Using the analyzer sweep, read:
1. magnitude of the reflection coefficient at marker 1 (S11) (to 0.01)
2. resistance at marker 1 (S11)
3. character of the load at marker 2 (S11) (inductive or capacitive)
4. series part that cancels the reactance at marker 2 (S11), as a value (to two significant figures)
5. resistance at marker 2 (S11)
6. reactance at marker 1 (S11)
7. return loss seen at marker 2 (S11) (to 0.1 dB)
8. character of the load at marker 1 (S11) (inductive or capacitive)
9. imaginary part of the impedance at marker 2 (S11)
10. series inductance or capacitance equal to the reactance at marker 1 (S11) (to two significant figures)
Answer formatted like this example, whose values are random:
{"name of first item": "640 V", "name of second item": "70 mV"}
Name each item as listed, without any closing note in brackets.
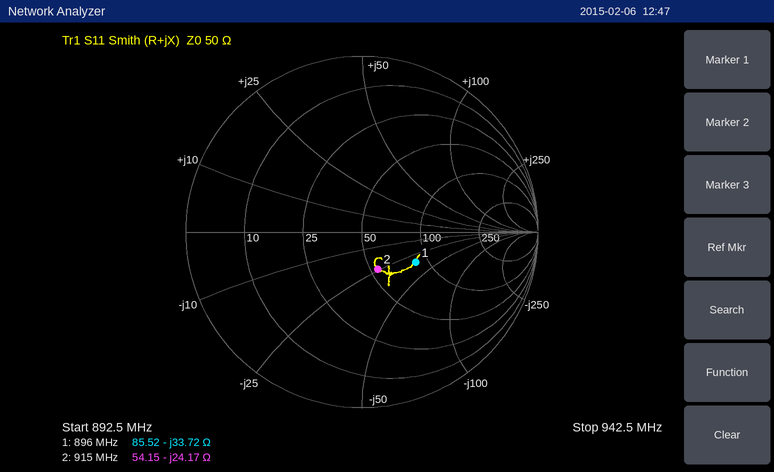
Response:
{"magnitude of the reflection coefficient at marker 1 (S11)": "0.35", "resistance at marker 1": "85.52 Ω", "character of the load at marker 2 (S11)": "capacitive", "series part that cancels the reactance at marker 2 (S11), as a value": "4.2 nH", "resistance at marker 2": "54.15 Ω", "reactance at marker 1": "-33.72 Ω", "return loss seen at marker 2 (S11)": "12.8 dB", "character of the load at marker 1 (S11)": "capacitive", "imaginary part of the impedance at marker 2": "-24.17 Ω", "series inductance or capacitance equal to the reactance at marker 1 (S11)": "5.3 pF"}
